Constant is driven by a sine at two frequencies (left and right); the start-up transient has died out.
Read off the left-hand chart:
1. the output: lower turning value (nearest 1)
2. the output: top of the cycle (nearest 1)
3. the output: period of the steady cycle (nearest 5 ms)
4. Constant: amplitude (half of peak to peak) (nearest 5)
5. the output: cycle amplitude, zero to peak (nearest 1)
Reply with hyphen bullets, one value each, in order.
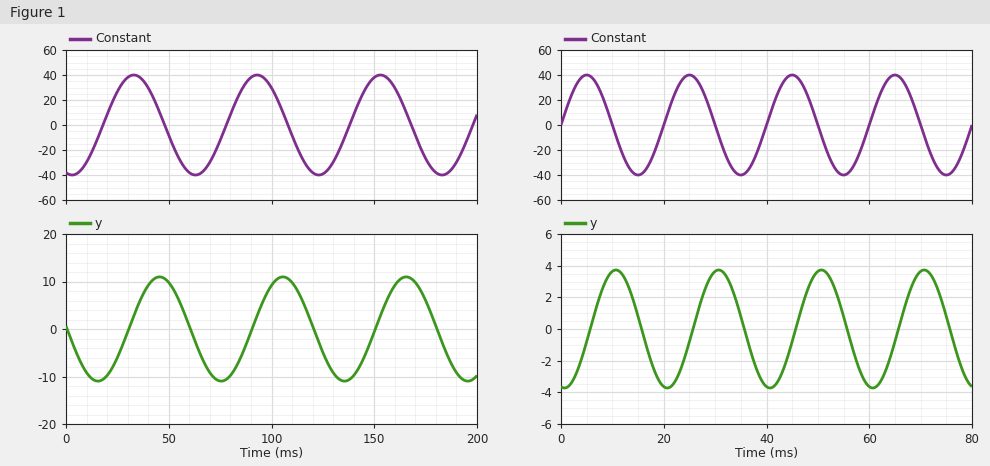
- -11
- 11
- 60 ms
- 40
- 11
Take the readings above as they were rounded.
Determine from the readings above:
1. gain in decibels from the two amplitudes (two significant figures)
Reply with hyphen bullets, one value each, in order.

- -11 dB
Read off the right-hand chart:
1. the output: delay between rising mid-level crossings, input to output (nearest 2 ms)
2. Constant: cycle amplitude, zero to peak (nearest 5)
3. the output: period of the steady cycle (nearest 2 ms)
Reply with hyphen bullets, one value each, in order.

- 6 ms
- 40
- 20 ms
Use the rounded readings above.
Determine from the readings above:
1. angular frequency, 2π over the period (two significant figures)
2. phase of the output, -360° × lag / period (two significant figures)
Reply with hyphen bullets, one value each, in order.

- 0.31 rad/ms
- -110°
